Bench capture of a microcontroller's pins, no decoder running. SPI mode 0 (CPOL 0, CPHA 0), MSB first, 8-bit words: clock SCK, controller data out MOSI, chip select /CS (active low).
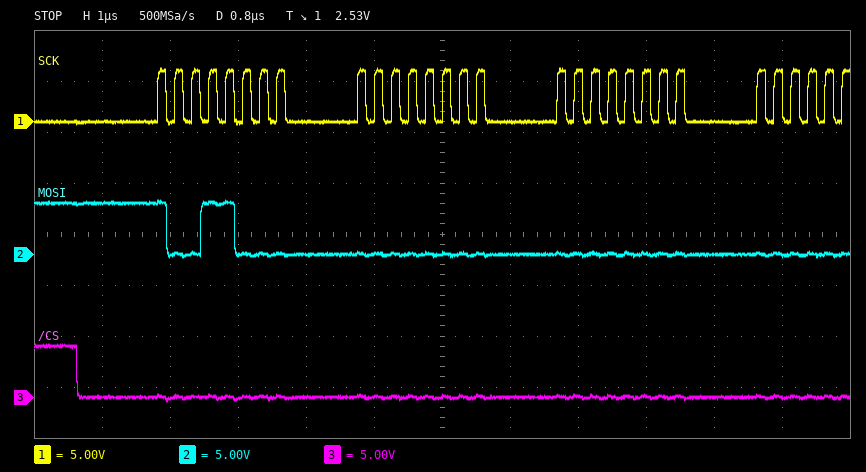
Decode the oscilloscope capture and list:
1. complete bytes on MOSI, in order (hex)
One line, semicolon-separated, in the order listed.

98 00 00
